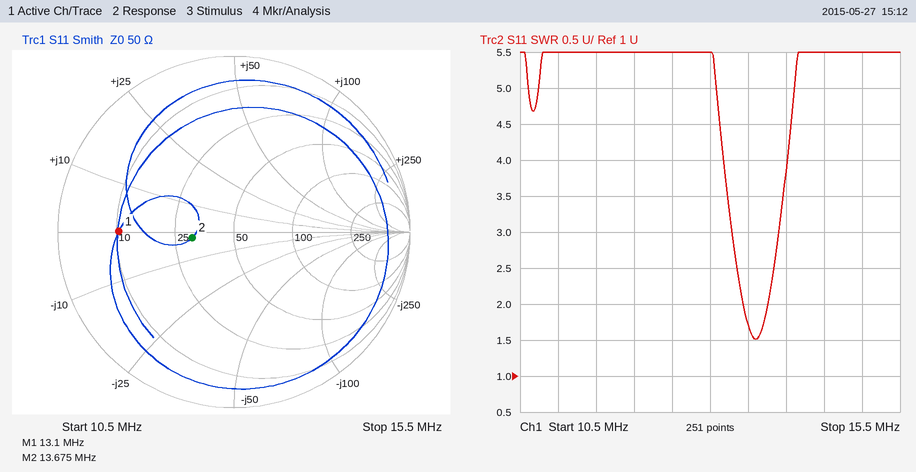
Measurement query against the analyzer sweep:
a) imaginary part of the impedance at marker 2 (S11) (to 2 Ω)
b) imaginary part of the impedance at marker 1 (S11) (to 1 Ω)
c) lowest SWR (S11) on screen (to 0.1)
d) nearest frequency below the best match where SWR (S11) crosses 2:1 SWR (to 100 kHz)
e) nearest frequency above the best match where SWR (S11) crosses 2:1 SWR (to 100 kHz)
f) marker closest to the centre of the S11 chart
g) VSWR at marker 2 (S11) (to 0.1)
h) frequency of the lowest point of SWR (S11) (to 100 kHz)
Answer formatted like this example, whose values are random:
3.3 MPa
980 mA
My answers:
-2 Ω
0 Ω
1.5
13.4 MHz
13.8 MHz
marker 2
1.6
13.6 MHz
